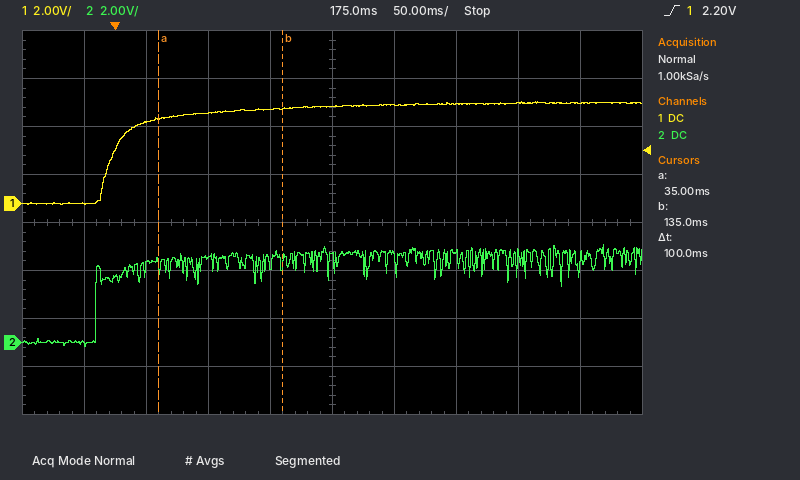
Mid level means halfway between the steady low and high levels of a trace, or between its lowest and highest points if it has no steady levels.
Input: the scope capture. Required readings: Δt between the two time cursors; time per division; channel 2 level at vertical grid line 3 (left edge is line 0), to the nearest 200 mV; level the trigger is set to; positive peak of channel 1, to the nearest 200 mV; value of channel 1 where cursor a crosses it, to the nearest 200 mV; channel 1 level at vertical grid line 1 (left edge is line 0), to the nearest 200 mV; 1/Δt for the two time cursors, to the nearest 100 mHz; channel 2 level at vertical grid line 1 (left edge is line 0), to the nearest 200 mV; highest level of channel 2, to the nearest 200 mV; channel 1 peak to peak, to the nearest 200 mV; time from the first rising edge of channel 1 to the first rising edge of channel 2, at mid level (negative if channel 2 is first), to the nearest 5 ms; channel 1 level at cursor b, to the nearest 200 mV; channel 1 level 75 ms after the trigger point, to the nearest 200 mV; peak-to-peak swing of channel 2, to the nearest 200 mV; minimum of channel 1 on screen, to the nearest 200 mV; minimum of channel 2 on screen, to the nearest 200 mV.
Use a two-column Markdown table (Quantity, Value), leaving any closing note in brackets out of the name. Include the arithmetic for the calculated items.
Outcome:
| Quantity | Value |
|---|---|
| Δt between the two time cursors | 100 ms |
| time per division | 50 ms |
| channel 2 level at vertical grid line 3 (left edge is line 0), to the nearest 200 mV | 3.6 V |
| level the trigger is set to | 2.20 V |
| positive peak of channel 1, to the nearest 200 mV | 4.2 V |
| value of channel 1 where cursor a crosses it, to the nearest 200 mV | 3.6 V |
| channel 1 level at vertical grid line 1 (left edge is line 0), to the nearest 200 mV | 0.0 V |
| 1/Δt for the two time cursors, to the nearest 100 mHz | 1 / 100 ms ≈ 10.0 Hz |
| channel 2 level at vertical grid line 1 (left edge is line 0), to the nearest 200 mV | 0.0 V |
| highest level of channel 2, to the nearest 200 mV | 4.0 V |
| channel 1 peak to peak, to the nearest 200 mV | 4.2 V − (0.0 V) = 4.2 V |
| time from the first rising edge of channel 1 to the first rising edge of channel 2, at mid level (negative if channel 2 is first), to the nearest 5 ms | -15 ms |
| channel 1 level at cursor b, to the nearest 200 mV | 4.0 V |
| channel 1 level 75 ms after the trigger point, to the nearest 200 mV | 3.8 V |
| peak-to-peak swing of channel 2, to the nearest 200 mV | 4.0 V − (-200 mV) = 4.2 V |
| minimum of channel 1 on screen, to the nearest 200 mV | 0.0 V |
| minimum of channel 2 on screen, to the nearest 200 mV | -200 mV |
